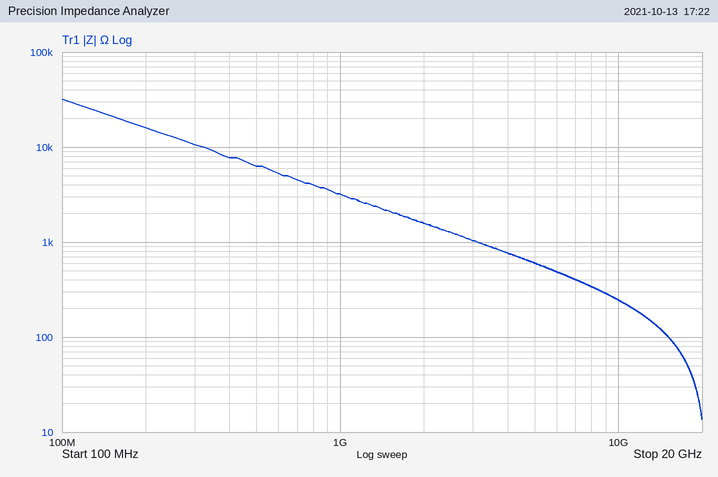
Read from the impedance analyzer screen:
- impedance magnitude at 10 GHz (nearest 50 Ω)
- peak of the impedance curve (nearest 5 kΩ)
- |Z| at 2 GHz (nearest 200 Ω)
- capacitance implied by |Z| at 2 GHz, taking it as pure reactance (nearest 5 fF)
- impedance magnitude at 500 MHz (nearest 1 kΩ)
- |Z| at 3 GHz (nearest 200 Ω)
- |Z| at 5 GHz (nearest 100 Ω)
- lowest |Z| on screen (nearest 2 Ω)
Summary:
250 Ω
30 kΩ
1.6 kΩ
50 fF
6 kΩ
1.0 kΩ
600 Ω
14 Ω
